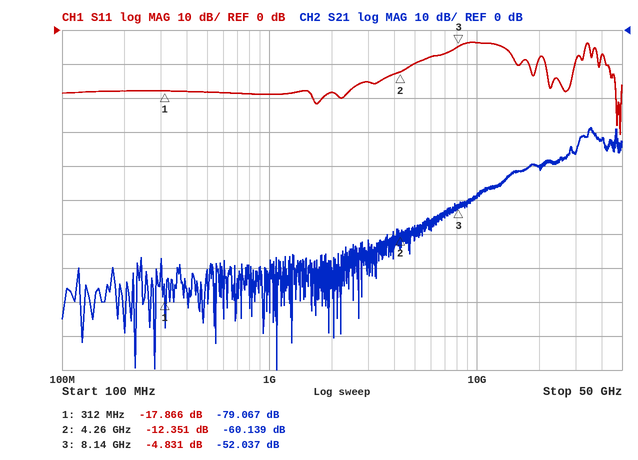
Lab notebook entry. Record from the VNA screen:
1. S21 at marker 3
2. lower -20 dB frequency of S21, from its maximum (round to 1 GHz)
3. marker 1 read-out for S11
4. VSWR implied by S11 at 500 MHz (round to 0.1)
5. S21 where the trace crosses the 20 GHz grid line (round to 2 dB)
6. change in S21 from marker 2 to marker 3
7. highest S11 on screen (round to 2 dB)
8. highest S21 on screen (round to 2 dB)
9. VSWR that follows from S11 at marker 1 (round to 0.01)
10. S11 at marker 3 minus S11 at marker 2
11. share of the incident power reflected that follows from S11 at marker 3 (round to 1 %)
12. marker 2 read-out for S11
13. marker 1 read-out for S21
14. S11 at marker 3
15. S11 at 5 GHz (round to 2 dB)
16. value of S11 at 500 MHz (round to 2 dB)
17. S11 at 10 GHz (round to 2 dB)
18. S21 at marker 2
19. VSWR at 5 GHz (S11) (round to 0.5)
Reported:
-52.037 dB
10 GHz
-17.866 dB
1.3
-40 dB
8.102 dB
-4 dB
-28 dB
1.29
7.520 dB
33 %
-12.351 dB
-79.067 dB
-4.831 dB
-10 dB
-18 dB
-4 dB
-60.139 dB
2.0
